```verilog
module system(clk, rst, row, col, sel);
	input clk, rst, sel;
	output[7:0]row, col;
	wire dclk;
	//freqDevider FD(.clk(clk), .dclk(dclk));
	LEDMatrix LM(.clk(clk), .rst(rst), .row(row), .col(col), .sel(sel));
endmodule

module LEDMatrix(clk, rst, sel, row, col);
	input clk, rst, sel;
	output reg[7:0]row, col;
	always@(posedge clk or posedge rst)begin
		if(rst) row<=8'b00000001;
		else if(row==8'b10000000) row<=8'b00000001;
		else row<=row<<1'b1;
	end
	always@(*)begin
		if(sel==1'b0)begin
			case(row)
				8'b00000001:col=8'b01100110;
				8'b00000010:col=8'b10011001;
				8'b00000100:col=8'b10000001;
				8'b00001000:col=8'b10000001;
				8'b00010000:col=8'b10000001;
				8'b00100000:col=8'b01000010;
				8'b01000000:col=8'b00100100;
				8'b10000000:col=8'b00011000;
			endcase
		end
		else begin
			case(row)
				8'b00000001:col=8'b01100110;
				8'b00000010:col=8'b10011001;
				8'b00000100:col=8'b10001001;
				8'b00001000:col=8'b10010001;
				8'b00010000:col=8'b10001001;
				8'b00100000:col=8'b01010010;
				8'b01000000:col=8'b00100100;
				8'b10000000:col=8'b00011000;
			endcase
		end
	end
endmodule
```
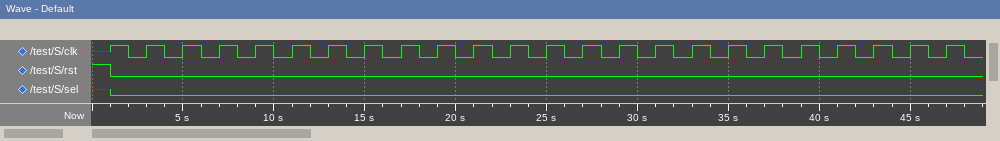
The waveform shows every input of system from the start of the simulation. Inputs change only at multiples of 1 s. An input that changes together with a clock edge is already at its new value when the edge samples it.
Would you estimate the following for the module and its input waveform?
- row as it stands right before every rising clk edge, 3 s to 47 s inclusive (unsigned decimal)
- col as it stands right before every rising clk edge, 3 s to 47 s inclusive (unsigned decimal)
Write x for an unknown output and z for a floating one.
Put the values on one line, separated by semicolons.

2, 4, 8, 16, 32, 64, 128, 1, 2, 4, 8, 16, 32, 64, 128, 1, 2, 4, 8, 16, 32, 64, 128; 153, 129, 129, 129, 66, 36, 24, 102, 153, 129, 129, 129, 66, 36, 24, 102, 153, 129, 129, 129, 66, 36, 24
